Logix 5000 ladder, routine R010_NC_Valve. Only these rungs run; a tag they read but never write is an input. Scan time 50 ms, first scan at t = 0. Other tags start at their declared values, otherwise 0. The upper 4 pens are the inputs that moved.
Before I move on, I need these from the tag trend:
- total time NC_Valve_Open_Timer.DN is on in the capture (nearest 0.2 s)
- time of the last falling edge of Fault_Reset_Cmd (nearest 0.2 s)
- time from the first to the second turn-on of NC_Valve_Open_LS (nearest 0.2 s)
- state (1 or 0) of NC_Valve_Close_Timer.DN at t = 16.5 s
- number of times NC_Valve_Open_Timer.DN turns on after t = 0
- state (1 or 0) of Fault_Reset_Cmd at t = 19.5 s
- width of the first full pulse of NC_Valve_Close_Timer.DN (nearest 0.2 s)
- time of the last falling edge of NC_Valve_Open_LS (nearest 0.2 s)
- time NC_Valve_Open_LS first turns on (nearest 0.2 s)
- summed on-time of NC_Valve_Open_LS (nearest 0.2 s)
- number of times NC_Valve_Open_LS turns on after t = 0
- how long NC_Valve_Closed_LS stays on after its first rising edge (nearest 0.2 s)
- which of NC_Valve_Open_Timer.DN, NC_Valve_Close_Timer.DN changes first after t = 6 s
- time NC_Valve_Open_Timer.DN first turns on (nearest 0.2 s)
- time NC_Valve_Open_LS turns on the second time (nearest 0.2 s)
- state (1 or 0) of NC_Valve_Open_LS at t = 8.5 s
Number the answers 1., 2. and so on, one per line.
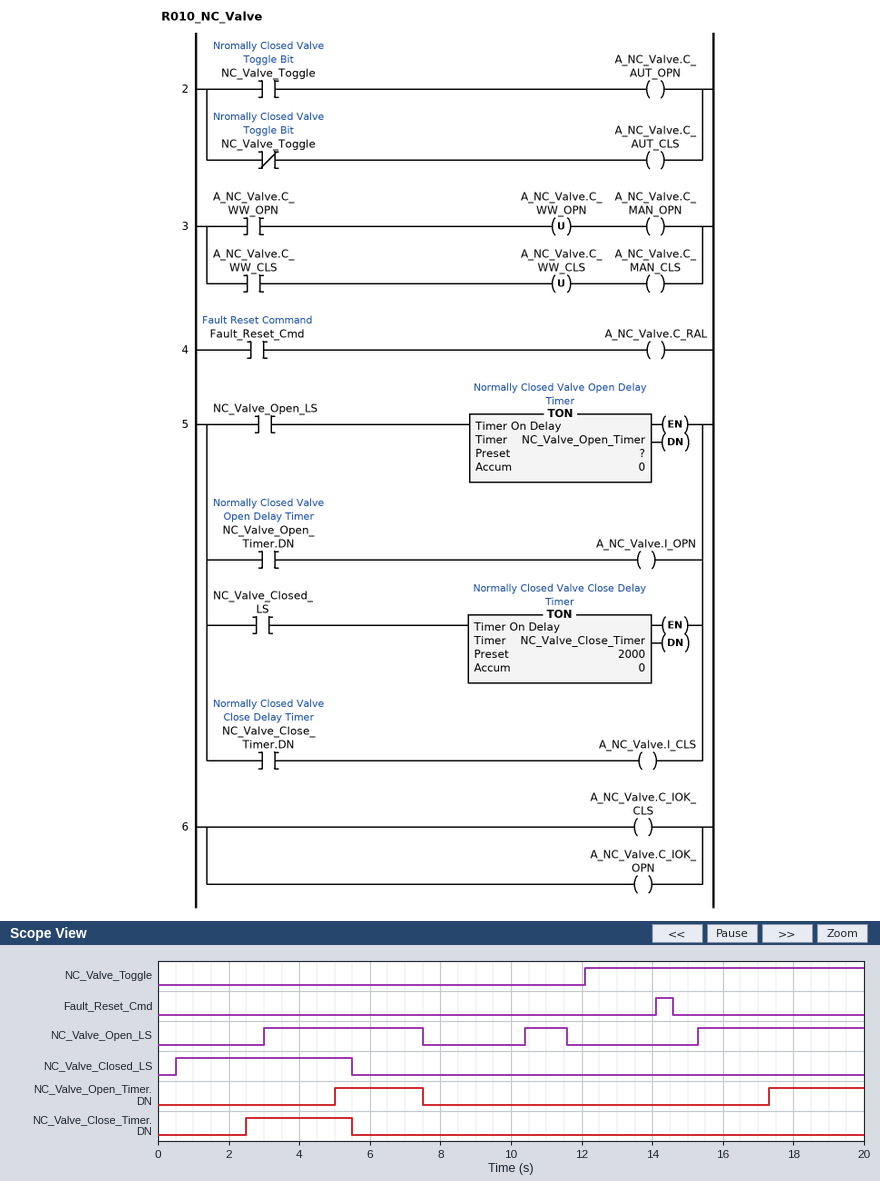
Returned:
1. 5.2 s
2. 14.6 s
3. 7.4 s
4. 0
5. 2
6. 0
7. 3.0 s
8. 11.6 s
9. 3.0 s
10. 10.4 s
11. 3
12. 5.0 s
13. NC_Valve_Open_Timer.DN
14. 5.0 s
15. 10.4 s
16. 0
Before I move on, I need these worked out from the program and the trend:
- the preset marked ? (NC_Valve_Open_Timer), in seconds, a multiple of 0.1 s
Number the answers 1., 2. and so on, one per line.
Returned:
1. 2.0 s
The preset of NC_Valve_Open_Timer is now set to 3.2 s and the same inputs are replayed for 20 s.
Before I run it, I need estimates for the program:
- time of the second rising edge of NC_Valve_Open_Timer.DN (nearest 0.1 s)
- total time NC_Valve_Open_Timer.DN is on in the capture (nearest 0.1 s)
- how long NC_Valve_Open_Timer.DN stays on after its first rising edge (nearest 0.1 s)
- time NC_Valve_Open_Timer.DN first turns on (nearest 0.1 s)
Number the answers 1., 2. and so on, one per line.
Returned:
1. 18.5 s
2. 2.8 s
3. 1.3 s
4. 6.2 s
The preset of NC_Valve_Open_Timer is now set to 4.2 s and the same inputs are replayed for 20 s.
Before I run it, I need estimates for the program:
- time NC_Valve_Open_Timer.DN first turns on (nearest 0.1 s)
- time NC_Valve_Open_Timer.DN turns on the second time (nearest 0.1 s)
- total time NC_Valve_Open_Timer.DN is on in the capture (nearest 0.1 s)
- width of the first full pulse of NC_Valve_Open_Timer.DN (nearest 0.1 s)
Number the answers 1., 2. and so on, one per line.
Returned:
1. 7.2 s
2. 19.5 s
3. 0.8 s
4. 0.3 s
